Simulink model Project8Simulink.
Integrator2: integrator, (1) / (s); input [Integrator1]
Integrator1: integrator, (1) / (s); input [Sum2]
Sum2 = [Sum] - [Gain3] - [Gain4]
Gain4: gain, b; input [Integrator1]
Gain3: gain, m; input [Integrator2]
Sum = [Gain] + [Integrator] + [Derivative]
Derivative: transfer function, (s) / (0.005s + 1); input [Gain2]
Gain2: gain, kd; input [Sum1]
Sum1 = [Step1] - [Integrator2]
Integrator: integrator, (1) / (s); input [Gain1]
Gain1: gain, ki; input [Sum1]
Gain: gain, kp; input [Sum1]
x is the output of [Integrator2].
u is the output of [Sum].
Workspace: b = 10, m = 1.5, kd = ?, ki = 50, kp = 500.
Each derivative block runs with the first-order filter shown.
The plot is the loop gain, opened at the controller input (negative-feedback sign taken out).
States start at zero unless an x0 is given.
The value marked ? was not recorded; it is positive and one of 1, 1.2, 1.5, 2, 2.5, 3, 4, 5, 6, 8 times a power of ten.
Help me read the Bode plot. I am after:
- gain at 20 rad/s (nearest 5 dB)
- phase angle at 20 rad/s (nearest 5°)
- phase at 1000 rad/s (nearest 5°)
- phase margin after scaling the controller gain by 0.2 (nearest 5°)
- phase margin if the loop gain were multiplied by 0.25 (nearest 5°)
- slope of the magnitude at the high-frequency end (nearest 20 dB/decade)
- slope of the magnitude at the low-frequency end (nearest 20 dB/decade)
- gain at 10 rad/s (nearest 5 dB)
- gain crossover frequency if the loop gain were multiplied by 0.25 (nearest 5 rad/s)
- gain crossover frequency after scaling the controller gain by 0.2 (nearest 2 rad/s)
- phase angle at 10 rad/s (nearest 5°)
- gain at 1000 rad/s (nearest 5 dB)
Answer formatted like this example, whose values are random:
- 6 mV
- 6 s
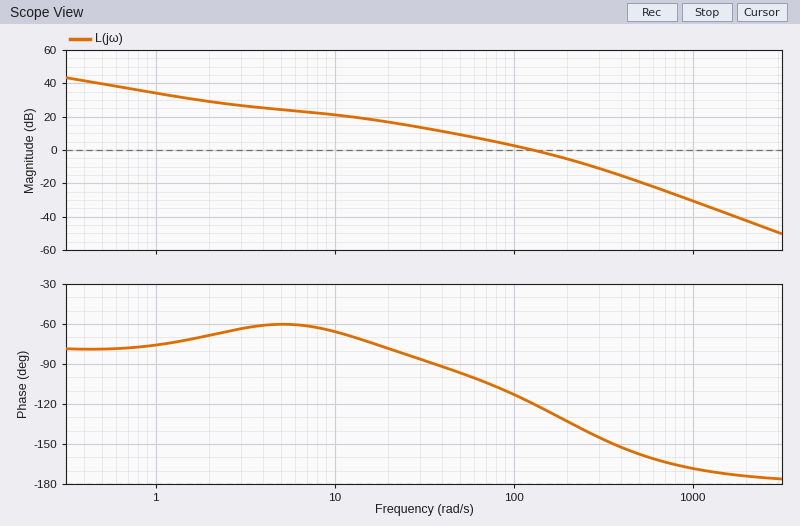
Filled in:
- 15 dB
- -80°
- -170°
- 95°
- 90°
- -40 dB/decade
- -20 dB/decade
- 20 dB
- 35 rad/s
- 28 rad/s
- -65°
- -30 dB
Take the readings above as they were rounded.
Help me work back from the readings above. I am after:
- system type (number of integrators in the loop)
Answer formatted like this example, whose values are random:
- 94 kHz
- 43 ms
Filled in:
- 1
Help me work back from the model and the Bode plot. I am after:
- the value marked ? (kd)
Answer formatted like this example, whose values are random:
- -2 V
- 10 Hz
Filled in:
- 150
